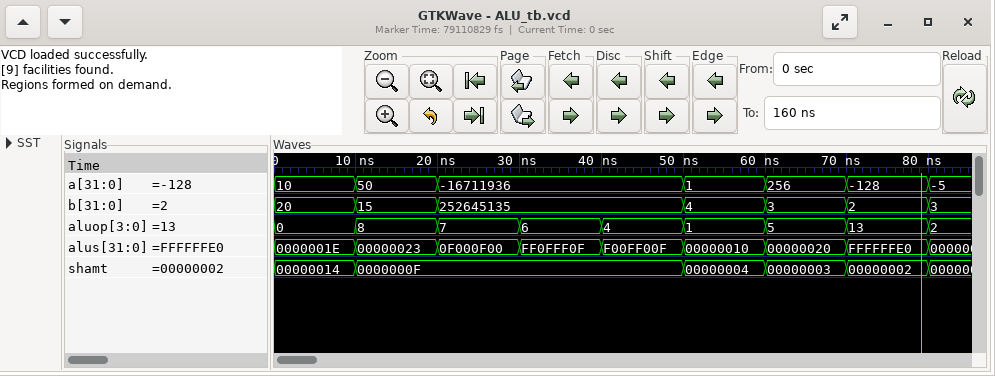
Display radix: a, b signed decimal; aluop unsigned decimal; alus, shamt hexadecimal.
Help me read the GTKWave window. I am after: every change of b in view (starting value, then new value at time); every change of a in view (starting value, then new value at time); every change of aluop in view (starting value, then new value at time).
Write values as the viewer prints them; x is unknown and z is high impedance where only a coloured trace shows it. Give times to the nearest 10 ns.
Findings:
20, 15 at 10 ns, 252645135 at 20 ns, 4 at 50 ns, 3 at 60 ns, 2 at 70 ns, 3 at 80 ns
10, 50 at 10 ns, -16711936 at 20 ns, 1 at 50 ns, 256 at 60 ns, -128 at 70 ns, -5 at 80 ns
0, 8 at 10 ns, 7 at 20 ns, 6 at 30 ns, 4 at 40 ns, 1 at 50 ns, 5 at 60 ns, 13 at 70 ns, 2 at 80 ns
